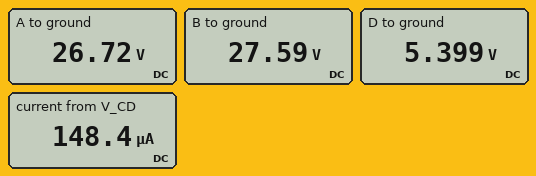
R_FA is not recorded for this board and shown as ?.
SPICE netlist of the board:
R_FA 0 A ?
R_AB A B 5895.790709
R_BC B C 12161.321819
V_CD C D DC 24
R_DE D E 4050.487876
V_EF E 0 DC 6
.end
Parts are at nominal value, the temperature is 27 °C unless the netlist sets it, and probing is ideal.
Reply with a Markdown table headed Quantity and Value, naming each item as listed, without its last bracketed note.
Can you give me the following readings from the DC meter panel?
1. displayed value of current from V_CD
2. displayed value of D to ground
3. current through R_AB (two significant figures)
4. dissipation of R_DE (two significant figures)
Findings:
| Quantity | Value |
|---|---|
| displayed value of current from V_CD | 148.4 µA |
| displayed value of D to ground | 5.399 V |
| current through R_AB | 150 µA |
| dissipation of R_DE | 89 µW |
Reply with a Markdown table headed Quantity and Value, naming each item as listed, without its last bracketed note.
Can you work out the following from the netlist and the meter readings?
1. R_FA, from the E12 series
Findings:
| Quantity | Value |
|---|---|
| R_FA, from the E12 series | 180 kΩ |
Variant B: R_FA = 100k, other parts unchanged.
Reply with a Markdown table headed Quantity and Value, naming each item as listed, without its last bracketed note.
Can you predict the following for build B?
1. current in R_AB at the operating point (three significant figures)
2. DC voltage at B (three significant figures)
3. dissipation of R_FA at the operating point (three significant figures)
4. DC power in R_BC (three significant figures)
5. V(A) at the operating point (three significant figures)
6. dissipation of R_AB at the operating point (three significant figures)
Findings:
| Quantity | Value |
|---|---|
| current in R_AB at the operating point | 246 µA |
| DC voltage at B | 26.0 V |
| dissipation of R_FA at the operating point | 6.04 mW |
| DC power in R_BC | 734 µW |
| V(A) at the operating point | 24.6 V |
| dissipation of R_AB at the operating point | 356 µW |
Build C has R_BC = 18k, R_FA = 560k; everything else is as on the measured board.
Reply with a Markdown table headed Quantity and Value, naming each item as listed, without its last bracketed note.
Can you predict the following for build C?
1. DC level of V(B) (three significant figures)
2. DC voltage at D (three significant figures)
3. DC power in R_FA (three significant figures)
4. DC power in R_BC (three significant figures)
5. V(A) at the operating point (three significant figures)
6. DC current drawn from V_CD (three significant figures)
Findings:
| Quantity | Value |
|---|---|
| DC level of V(B) | 28.9 V |
| DC voltage at D | 5.79 V |
| DC power in R_FA | 1.46 mW |
| DC power in R_BC | 46.9 µW |
| V(A) at the operating point | 28.6 V |
| DC current drawn from V_CD | 51.0 µA |
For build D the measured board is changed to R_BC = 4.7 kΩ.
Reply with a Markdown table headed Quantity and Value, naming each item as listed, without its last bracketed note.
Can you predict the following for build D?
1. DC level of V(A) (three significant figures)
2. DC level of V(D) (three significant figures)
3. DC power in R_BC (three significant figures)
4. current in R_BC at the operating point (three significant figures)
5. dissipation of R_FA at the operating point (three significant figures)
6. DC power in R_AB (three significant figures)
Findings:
| Quantity | Value |
|---|---|
| DC level of V(A) | 27.7 V |
| DC level of V(D) | 5.38 V |
| DC power in R_BC | 112 µW |
| current in R_BC at the operating point | 154 µA |
| dissipation of R_FA at the operating point | 4.28 mW |
| DC power in R_AB | 140 µW |
